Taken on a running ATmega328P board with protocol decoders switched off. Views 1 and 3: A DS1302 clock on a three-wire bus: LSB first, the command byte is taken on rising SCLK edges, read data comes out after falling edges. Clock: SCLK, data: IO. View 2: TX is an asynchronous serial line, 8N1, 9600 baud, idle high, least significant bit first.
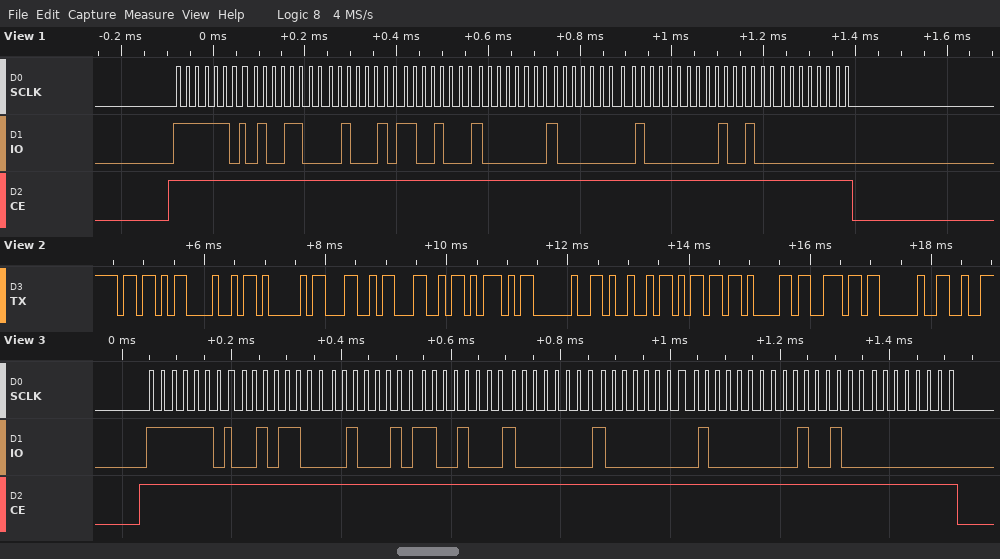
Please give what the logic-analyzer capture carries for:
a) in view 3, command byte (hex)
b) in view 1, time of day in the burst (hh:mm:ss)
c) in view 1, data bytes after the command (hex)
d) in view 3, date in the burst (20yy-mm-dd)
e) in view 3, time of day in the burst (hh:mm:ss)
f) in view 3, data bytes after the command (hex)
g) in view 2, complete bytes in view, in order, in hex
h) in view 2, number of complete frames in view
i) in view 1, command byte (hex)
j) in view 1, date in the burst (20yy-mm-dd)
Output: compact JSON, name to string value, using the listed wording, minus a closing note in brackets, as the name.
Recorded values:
{"in view 3, command byte": "0xBF", "in view 1, time of day in the burst": "13:44:32", "in view 1, data bytes after the command": "32 44 13 01 01 02 24 00", "in view 3, date in the burst": "2024-01-01", "in view 3, time of day in the burst": "13:44:34", "in view 3, data bytes after the command": "34 44 13 01 01 02 24 00", "in view 2, complete bytes in view, in order, in hex": "5B 48 41 4C 4C 5D 20 49 6D 61 6E 20", "in view 2, number of complete frames in view": "12", "in view 1, command byte": "0xBF", "in view 1, date in the burst": "2024-01-01"}
